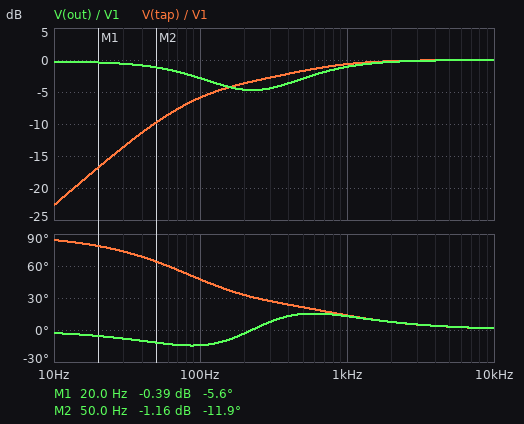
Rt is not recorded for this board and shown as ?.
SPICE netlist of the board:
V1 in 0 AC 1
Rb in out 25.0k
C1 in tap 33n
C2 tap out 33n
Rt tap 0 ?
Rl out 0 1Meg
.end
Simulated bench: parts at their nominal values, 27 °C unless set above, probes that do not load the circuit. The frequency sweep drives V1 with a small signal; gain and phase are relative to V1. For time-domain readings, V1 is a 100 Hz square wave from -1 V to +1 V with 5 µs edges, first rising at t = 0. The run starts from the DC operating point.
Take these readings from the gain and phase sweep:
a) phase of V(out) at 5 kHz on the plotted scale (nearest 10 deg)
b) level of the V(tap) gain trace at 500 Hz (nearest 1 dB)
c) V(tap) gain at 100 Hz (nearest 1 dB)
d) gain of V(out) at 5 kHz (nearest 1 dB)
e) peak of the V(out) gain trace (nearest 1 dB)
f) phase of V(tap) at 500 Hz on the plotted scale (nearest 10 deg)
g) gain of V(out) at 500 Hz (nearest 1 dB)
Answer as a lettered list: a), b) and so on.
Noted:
a) 0 deg
b) -2 dB
c) -6 dB
d) 0 dB
e) 0 dB
f) 20 deg
g) -3 dB
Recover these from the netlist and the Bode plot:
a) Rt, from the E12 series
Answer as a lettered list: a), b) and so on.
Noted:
a) 18 kΩ
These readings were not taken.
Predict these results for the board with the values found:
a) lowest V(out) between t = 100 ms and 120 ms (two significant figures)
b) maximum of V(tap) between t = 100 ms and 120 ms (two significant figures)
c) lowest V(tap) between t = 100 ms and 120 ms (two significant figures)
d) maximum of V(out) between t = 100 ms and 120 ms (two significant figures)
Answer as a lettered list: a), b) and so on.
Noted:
a) -1.1 V
b) 1.9 V
c) -1.9 V
d) 1.1 V
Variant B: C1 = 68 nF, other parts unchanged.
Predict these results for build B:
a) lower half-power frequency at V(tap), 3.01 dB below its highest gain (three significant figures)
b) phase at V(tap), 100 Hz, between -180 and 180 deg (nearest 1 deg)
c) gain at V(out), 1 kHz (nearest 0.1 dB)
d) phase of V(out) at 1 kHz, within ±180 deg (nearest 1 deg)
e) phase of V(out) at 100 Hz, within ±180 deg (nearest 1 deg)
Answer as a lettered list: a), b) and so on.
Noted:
a) 111 Hz
b) 39 deg
c) -0.4 dB
d) 7 deg
e) -7 deg
